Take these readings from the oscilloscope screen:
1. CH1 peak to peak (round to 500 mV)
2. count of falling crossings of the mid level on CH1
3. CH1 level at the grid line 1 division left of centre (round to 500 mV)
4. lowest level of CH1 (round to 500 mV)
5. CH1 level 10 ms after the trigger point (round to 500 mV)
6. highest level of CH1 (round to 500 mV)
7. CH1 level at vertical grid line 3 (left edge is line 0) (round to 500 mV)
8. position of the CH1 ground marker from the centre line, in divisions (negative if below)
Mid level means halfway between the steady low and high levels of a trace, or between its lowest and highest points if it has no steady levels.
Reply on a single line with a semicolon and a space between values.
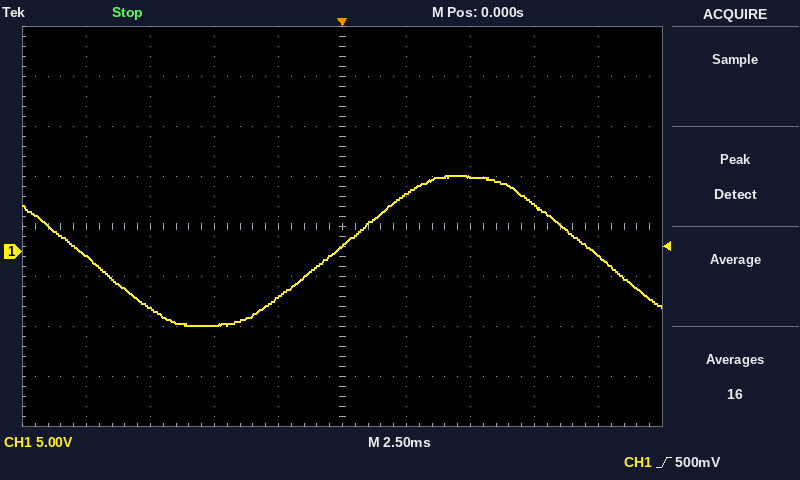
15.0 V; 2; -4.5 V; -7.5 V; -500 mV; 7.5 V; -7.5 V; -0.5 div
